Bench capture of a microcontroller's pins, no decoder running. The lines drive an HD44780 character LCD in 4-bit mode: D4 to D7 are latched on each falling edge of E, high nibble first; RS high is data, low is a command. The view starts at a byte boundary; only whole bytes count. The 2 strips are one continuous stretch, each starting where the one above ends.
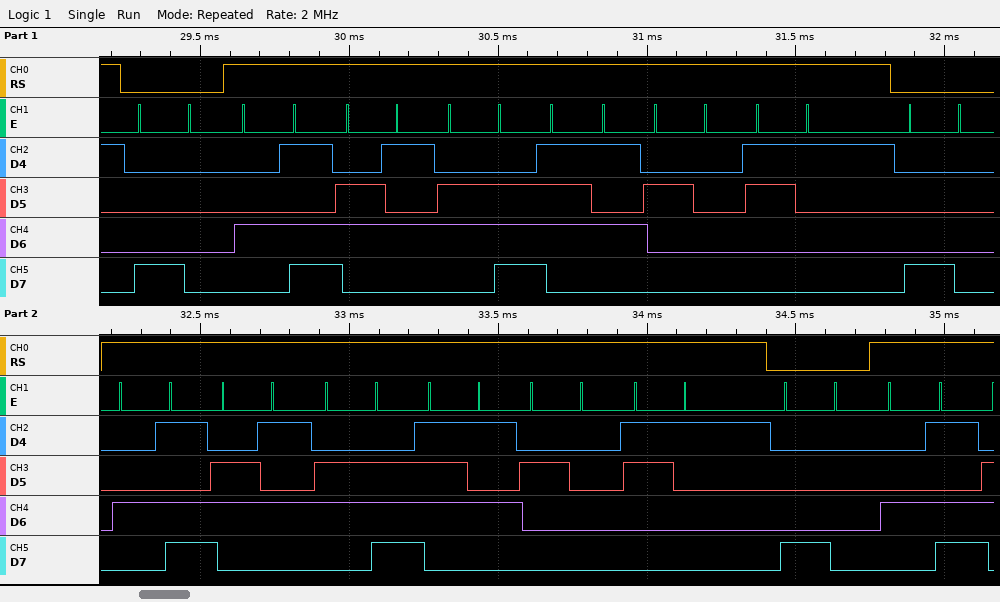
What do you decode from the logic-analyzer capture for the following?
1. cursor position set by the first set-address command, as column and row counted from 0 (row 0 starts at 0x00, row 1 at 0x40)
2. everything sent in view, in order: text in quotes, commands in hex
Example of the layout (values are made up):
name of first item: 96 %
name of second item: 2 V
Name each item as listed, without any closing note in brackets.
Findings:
cursor position set by the first set-address command, as column and row counted from 0: column 0, row 0
everything sent in view, in order: text in quotes, commands in hex: 0x80 "Menu 1" 0x80 "Menu 1" 0x80 "M"
